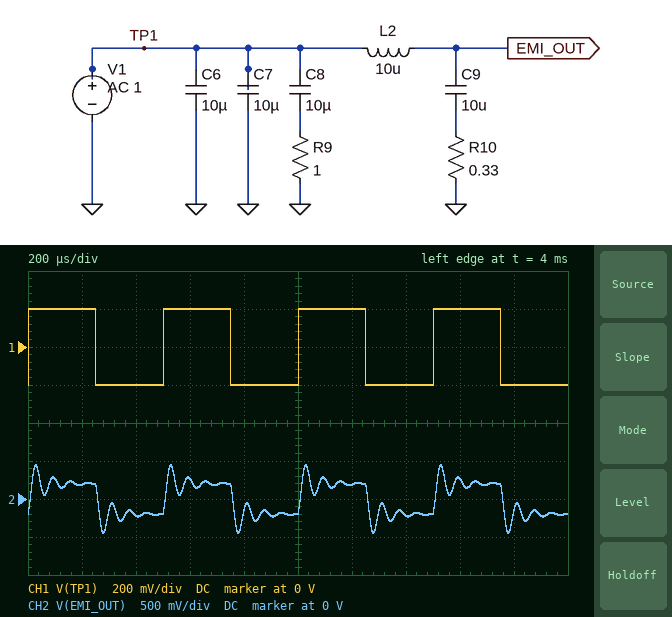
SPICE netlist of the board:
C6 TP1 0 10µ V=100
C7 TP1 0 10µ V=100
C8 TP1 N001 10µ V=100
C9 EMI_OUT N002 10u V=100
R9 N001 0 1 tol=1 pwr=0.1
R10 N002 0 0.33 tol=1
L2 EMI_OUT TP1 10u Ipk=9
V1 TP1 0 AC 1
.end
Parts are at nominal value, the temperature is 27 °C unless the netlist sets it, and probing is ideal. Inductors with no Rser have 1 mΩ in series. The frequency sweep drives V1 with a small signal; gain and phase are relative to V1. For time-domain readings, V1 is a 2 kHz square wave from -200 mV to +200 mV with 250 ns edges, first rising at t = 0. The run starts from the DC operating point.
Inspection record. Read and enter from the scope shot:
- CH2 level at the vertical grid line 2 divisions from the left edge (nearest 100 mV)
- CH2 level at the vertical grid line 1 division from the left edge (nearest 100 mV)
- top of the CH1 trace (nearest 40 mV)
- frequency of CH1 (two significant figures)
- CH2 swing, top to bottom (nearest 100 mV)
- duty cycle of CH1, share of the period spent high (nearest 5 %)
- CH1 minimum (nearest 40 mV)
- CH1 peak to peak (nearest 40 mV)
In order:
-200 mV
200 mV
200 mV
2.0 kHz
900 mV
50 %
-200 mV
400 mV
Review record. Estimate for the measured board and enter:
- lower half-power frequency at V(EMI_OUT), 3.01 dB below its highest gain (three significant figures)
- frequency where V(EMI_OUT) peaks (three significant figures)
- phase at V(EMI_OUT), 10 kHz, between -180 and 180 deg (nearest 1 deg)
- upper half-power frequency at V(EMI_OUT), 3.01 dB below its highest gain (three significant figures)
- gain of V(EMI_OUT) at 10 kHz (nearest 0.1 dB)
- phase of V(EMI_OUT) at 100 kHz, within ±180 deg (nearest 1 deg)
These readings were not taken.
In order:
12.6 kHz
15.5 kHz
-7 deg
18.0 kHz
4.1 dB
-113 deg
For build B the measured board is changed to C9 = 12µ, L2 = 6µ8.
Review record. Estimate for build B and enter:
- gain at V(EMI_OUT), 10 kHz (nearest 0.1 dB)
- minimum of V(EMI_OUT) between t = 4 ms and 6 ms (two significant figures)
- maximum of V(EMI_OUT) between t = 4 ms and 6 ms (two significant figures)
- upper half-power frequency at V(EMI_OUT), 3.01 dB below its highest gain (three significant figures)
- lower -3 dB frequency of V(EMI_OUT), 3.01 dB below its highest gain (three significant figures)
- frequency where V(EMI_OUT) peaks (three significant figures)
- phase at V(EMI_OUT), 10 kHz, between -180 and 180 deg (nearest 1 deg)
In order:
3.1 dB
-420 mV
420 mV
20.6 kHz
12.5 kHz
16.9 kHz
-6 deg
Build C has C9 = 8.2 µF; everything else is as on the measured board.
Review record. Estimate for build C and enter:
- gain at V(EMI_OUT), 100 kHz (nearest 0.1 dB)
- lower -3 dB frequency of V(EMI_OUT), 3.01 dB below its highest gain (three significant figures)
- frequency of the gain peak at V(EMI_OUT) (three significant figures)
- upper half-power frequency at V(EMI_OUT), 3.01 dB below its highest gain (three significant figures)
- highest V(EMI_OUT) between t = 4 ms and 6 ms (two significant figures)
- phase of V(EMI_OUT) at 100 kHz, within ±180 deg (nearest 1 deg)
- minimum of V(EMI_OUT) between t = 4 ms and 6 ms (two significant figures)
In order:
-24.0 dB
14.3 kHz
17.2 kHz
19.7 kHz
460 mV
-117 deg
-460 mV
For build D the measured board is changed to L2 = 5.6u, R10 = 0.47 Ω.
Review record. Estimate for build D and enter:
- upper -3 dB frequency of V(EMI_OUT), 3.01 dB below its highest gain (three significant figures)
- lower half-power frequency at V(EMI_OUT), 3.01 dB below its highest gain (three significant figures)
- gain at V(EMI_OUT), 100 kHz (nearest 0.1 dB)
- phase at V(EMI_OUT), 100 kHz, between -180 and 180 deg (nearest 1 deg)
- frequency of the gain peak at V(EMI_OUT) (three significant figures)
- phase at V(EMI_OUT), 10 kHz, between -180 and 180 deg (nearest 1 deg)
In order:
26.1 kHz
11.8 kHz
-16.7 dB
-101 deg
19.7 kHz
-4 deg
